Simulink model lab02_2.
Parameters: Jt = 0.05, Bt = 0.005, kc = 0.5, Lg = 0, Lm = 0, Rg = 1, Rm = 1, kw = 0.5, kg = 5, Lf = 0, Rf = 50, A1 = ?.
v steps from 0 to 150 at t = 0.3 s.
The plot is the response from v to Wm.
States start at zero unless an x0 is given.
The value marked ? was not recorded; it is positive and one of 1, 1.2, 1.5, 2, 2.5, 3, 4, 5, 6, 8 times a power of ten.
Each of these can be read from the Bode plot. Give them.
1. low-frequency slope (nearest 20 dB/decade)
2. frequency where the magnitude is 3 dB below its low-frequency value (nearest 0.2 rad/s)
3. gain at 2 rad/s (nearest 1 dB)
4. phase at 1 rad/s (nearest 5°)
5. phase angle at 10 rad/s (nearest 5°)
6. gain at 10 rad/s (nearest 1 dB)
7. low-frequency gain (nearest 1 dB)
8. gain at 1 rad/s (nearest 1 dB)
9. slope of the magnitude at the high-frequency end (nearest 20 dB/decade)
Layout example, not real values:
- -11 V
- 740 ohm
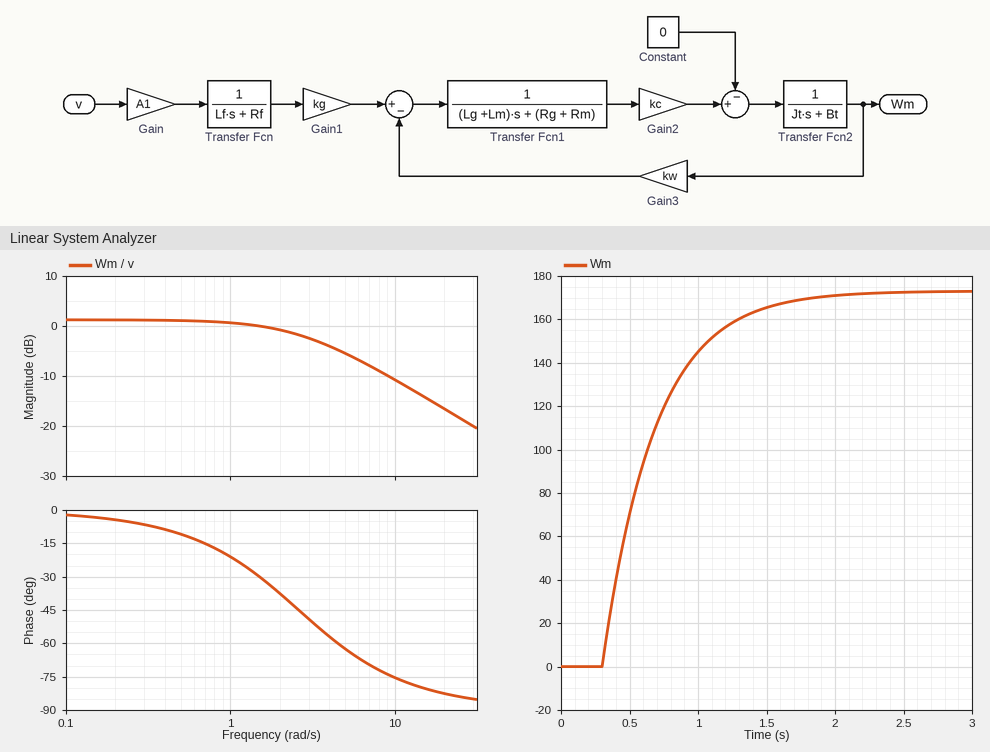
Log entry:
- 0 dB/decade
- 2.6 rad/s
- -1 dB
- -20°
- -75°
- -11 dB
- 1 dB
- 1 dB
- -20 dB/decade
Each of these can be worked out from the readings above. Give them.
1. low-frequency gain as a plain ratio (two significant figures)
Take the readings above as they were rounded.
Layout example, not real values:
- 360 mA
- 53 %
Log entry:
- 1.1
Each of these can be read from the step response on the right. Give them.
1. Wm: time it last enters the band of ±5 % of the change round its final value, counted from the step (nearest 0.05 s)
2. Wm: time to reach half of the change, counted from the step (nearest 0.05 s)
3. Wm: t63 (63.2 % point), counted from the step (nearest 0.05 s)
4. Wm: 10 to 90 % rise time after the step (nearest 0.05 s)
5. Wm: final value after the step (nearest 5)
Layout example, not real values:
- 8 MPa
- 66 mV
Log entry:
- 1.15 s
- 0.25 s
- 0.40 s
- 0.85 s
- 175
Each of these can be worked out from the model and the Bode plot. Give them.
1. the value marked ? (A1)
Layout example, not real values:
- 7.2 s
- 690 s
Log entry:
- 6
